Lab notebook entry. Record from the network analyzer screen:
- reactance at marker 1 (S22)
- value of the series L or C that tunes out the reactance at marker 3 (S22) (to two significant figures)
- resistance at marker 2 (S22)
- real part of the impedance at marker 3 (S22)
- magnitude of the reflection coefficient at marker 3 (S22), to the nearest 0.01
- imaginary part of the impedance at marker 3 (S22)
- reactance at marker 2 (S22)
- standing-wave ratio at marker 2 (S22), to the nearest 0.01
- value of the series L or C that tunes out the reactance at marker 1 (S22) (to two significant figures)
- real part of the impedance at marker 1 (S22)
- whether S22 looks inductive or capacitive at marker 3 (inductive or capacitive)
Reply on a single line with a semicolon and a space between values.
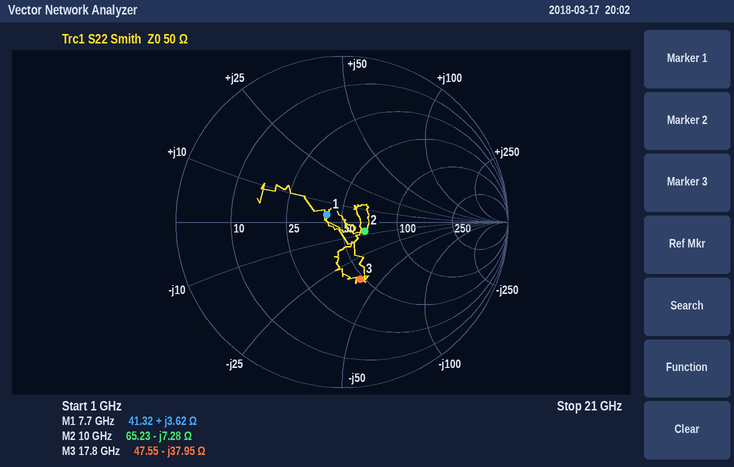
+3.62 Ω; 340 pH; 65.23 Ω; 47.55 Ω; 0.36; -37.95 Ω; -7.28 Ω; 1.34; 5.7 pF; 41.32 Ω; capacitive
